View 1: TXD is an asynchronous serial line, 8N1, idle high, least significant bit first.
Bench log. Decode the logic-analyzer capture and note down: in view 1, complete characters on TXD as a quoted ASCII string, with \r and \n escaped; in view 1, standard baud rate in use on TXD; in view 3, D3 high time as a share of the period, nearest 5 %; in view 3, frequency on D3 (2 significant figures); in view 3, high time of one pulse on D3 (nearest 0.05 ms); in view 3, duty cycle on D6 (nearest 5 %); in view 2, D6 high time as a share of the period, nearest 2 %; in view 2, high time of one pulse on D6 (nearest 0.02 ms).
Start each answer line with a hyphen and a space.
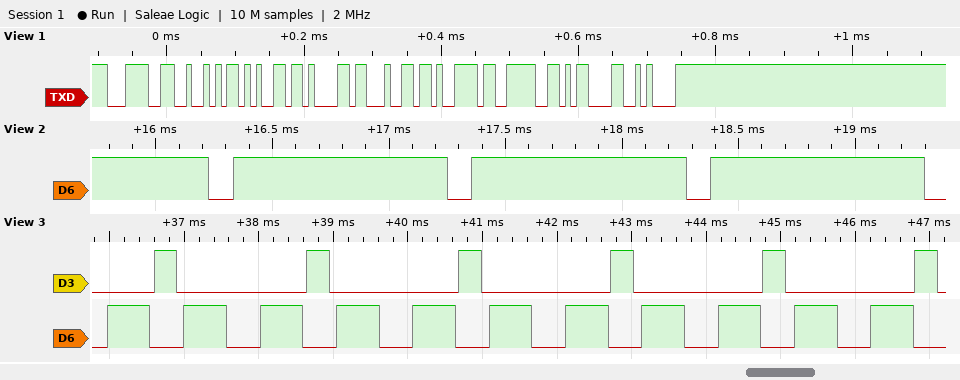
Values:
- "<Ready>\r\n"
- 115200 baud
- 15 %
- 490 Hz
- 0.30 ms
- 55 %
- 90 %
- 0.92 ms
